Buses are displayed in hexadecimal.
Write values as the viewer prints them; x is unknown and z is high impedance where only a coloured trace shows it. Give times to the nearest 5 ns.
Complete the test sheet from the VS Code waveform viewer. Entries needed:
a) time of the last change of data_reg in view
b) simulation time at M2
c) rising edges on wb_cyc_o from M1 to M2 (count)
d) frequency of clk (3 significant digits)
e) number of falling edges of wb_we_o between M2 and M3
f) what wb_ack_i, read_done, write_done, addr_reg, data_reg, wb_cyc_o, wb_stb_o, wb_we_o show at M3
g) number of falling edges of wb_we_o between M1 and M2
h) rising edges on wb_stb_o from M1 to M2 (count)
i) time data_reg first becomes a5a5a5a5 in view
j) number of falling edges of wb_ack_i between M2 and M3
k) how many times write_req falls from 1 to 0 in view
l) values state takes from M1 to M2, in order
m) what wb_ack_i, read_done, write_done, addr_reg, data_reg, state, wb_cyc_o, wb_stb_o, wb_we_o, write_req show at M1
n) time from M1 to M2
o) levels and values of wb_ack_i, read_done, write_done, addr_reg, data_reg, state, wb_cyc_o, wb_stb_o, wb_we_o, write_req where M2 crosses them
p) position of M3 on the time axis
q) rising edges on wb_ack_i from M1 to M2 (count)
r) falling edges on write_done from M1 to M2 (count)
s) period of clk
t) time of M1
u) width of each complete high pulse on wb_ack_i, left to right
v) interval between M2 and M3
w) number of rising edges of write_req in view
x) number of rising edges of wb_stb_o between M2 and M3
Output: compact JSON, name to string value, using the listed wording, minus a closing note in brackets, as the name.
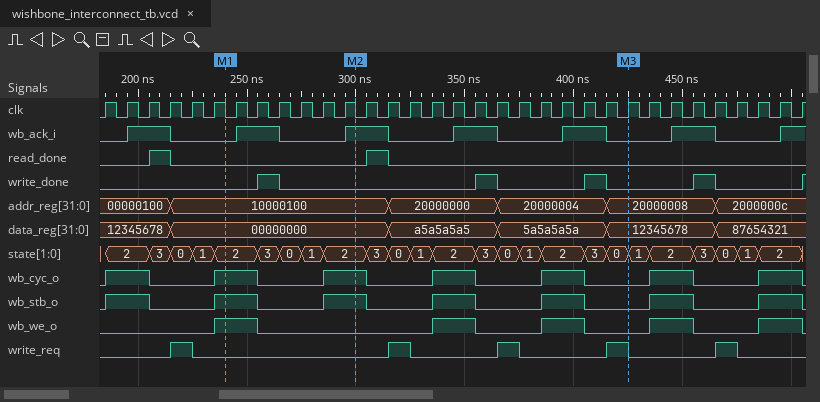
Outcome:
{"time of the last change of data_reg in view": "465 ns", "simulation time at M2": "300 ns", "rising edges on wb_cyc_o from M1 to M2": "1", "frequency of clk": "100 MHz", "number of falling edges of wb_we_o between M2 and M3": "2", "what wb_ack_i, read_done, write_done, addr_reg, data_reg, wb_cyc_o, wb_stb_o, wb_we_o show at M3": "wb_ack_i=0, read_done=0, write_done=0, addr_reg=20000008, data_reg=12345678, wb_cyc_o=0, wb_stb_o=0, wb_we_o=0", "number of falling edges of wb_we_o between M1 and M2": "1", "rising edges on wb_stb_o from M1 to M2": "1", "time data_reg first becomes a5a5a5a5 in view": "315 ns", "number of falling edges of wb_ack_i between M2 and M3": "3", "how many times write_req falls from 1 to 0 in view": "5", "values state takes from M1 to M2, in order": "2, 3, 0, 1, 2", "what wb_ack_i, read_done, write_done, addr_reg, data_reg, state, wb_cyc_o, wb_stb_o, wb_we_o, write_req show at M1": "wb_ack_i=0, read_done=0, write_done=0, addr_reg=10000100, data_reg=00000000, state=2, wb_cyc_o=1, wb_stb_o=1, wb_we_o=1, write_req=0", "time from M1 to M2": "60 ns", "levels and values of wb_ack_i, read_done, write_done, addr_reg, data_reg, state, wb_cyc_o, wb_stb_o, wb_we_o, write_req where M2 crosses them": "wb_ack_i=1, read_done=0, write_done=0, addr_reg=10000100, data_reg=00000000, state=2, wb_cyc_o=1, wb_stb_o=1, wb_we_o=0, write_req=0", "position of M3 on the time axis": "425 ns", "rising edges on wb_ack_i from M1 to M2": "2", "falling edges on write_done from M1 to M2": "1", "period of clk": "10 ns", "time of M1": "240 ns", "width of each complete high pulse on wb_ack_i, left to right": "20 ns, 20 ns, 20 ns, 20 ns, 20 ns, 20 ns", "interval between M2 and M3": "125 ns", "number of rising edges of write_req in view": "5", "number of rising edges of wb_stb_o between M2 and M3": "2"}
